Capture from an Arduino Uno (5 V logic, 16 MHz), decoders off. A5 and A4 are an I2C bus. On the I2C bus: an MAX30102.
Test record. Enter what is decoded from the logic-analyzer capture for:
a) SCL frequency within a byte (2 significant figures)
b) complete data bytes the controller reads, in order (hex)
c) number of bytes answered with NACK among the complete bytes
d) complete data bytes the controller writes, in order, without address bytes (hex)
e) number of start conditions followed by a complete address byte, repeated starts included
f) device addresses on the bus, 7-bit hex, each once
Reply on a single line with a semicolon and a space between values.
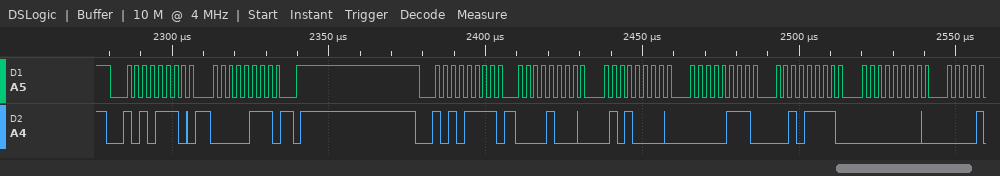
400 kHz; 08 50 07 2F 00; 0; 07; 2; 0x57
